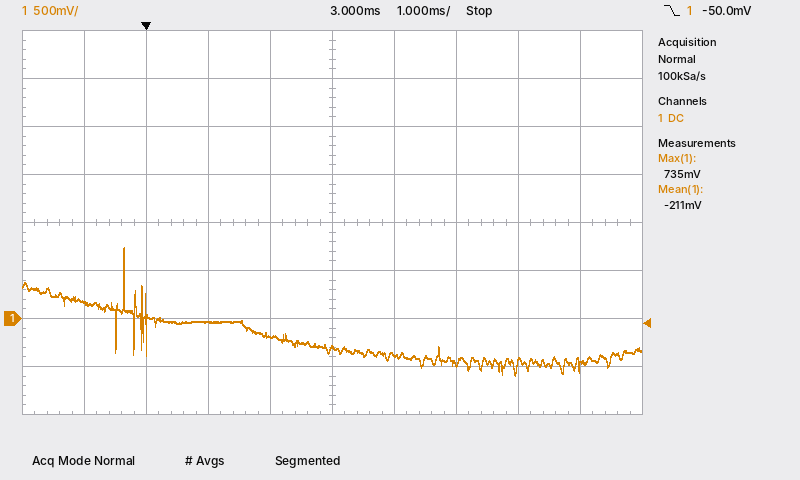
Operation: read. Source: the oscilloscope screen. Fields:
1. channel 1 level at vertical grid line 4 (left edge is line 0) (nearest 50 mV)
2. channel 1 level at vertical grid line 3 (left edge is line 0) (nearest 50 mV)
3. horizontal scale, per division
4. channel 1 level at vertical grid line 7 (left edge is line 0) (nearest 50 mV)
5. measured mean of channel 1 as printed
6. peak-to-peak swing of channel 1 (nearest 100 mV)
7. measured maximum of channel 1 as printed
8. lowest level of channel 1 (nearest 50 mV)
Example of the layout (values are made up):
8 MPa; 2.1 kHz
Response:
-200 mV; -50 mV; 1 ms; -450 mV; -211 mV; 1.30 V; 735 mV; -600 mV
